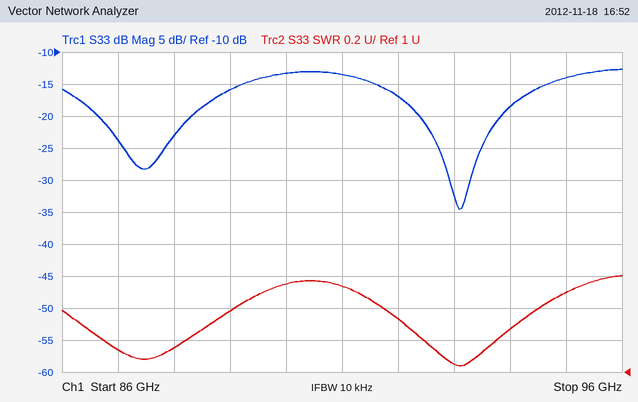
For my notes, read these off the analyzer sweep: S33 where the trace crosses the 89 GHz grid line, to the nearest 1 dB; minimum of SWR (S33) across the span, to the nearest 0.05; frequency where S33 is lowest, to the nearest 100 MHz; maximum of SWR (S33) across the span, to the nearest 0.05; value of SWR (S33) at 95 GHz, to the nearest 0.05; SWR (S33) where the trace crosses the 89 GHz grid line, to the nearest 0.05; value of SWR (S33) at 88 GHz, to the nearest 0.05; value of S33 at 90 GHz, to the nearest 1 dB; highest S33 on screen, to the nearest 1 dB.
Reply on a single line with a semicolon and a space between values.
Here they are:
-16 dB; 1.05; 93.1 GHz; 1.60; 1.50; 1.40; 1.15; -13 dB; -13 dB
